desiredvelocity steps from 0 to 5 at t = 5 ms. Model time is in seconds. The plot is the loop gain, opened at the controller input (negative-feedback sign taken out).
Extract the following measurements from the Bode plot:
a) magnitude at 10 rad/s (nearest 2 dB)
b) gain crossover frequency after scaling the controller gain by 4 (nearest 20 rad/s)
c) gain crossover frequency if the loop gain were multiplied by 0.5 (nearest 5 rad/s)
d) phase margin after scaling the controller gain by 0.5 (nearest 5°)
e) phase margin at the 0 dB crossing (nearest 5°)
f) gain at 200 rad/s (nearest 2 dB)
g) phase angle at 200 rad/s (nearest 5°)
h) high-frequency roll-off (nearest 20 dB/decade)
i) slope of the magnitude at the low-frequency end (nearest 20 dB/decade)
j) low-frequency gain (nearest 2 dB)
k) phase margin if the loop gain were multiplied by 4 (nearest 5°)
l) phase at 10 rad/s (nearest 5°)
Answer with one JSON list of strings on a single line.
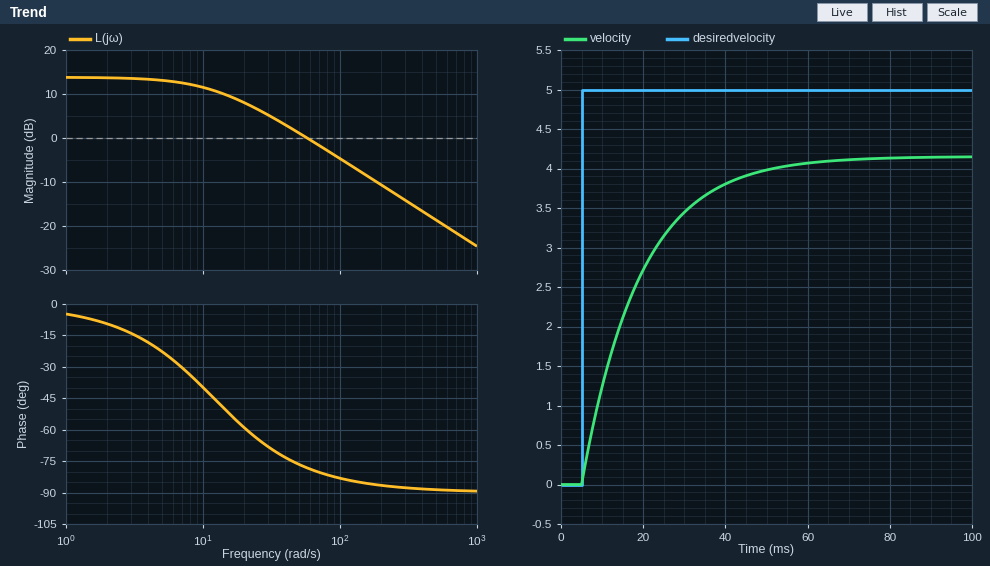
["12 dB", "240 rad/s", "25 rad/s", "115°", "100°", "-10 dB", "-85°", "-20 dB/decade", "0 dB/decade", "14 dB", "95°", "-40°"]
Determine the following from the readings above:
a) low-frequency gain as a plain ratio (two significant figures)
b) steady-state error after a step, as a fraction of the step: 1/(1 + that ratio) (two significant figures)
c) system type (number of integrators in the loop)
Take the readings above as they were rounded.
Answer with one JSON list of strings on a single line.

["5.0", "0.17", "0"]
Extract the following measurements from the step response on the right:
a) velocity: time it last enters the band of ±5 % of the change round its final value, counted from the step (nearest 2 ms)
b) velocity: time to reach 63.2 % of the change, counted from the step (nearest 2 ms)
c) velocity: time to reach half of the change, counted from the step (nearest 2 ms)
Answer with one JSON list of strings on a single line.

["42 ms", "14 ms", "10 ms"]
